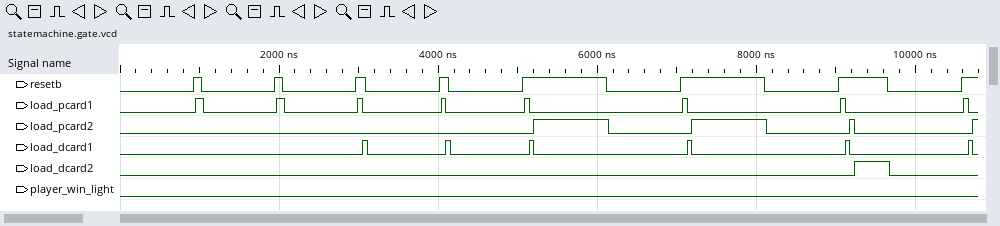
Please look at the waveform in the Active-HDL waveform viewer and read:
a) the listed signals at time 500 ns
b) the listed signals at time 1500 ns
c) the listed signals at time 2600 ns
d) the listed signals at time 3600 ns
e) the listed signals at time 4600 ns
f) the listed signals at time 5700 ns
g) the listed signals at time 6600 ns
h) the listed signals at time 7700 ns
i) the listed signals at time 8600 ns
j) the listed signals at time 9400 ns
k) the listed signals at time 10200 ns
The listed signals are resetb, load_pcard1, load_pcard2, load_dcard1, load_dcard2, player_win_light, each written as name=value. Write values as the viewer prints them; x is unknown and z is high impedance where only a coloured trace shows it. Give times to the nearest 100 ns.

resetb=0, load_pcard1=0, load_pcard2=0, load_dcard1=0, load_dcard2=0, player_win_light=0
resetb=0, load_pcard1=0, load_pcard2=0, load_dcard1=0, load_dcard2=0, player_win_light=0
resetb=0, load_pcard1=0, load_pcard2=0, load_dcard1=0, load_dcard2=0, player_win_light=0
resetb=0, load_pcard1=0, load_pcard2=0, load_dcard1=0, load_dcard2=0, player_win_light=0
resetb=0, load_pcard1=0, load_pcard2=0, load_dcard1=0, load_dcard2=0, player_win_light=0
resetb=1, load_pcard1=0, load_pcard2=1, load_dcard1=0, load_dcard2=0, player_win_light=0
resetb=0, load_pcard1=0, load_pcard2=0, load_dcard1=0, load_dcard2=0, player_win_light=0
resetb=1, load_pcard1=0, load_pcard2=1, load_dcard1=0, load_dcard2=0, player_win_light=0
resetb=0, load_pcard1=0, load_pcard2=0, load_dcard1=0, load_dcard2=0, player_win_light=0
resetb=1, load_pcard1=0, load_pcard2=0, load_dcard1=0, load_dcard2=1, player_win_light=0
resetb=0, load_pcard1=0, load_pcard2=0, load_dcard1=0, load_dcard2=0, player_win_light=0
